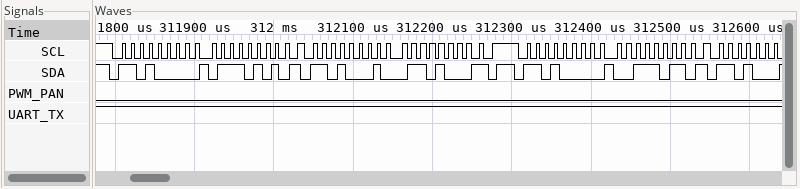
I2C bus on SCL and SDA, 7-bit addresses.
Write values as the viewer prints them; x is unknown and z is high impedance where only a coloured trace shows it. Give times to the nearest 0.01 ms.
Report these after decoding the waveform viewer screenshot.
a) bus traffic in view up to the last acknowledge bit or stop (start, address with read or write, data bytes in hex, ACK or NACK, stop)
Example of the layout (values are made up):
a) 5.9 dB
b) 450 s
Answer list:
a) start, address 68 write ACK, 75 ACK, repeated start, address 68 read ACK, 68 NACK, stop, start, address 68 write ACK, 3B ACK
